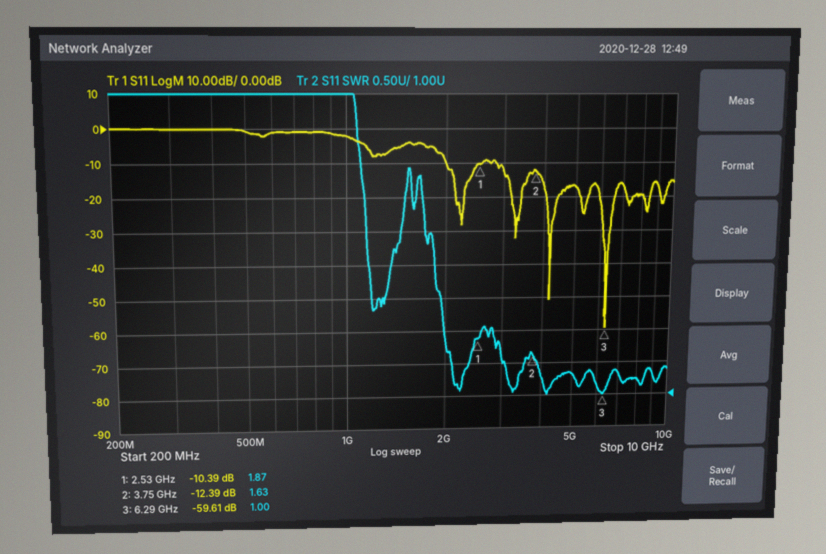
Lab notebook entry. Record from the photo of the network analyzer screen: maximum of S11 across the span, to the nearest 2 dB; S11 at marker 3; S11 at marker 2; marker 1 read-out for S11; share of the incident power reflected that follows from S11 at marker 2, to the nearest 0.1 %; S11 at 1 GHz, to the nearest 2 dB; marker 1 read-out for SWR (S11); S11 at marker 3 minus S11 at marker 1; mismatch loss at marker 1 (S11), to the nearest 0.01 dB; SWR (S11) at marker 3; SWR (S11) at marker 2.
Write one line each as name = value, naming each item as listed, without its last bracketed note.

maximum of S11 across the span, to the nearest 2 dB = 0 dB
S11 at marker 3 = -59.61 dB
S11 at marker 2 = -12.39 dB
marker 1 read-out for S11 = -10.39 dB
share of the incident power reflected that follows from S11 at marker 2, to the nearest 0.1 % = 5.8 %
S11 at 1 GHz, to the nearest 2 dB = -2 dB
marker 1 read-out for SWR = 1.87
S11 at marker 3 minus S11 at marker 1 = -49.22 dB
mismatch loss at marker 1 (S11), to the nearest 0.01 dB = 0.42 dB
SWR (S11) at marker 3 = 1.00
SWR (S11) at marker 2 = 1.63
